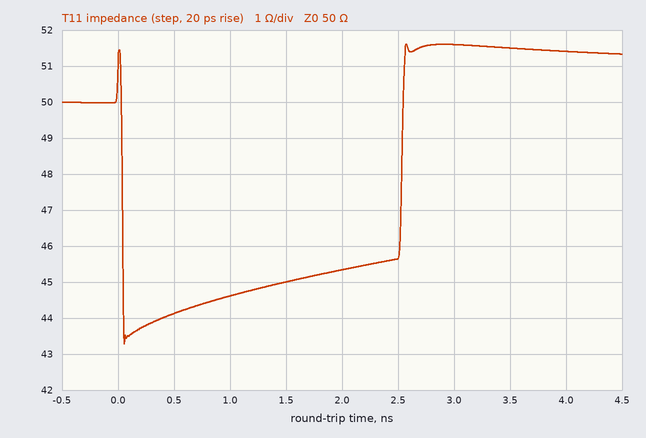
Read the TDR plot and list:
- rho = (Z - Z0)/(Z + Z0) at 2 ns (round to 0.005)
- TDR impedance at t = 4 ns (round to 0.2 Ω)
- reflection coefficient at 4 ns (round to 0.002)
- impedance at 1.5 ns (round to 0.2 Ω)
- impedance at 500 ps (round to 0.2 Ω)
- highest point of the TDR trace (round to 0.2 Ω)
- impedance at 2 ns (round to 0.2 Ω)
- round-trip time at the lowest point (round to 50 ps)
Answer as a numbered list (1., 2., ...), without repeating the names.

1. -0.050
2. 51.4 Ω
3. +0.014
4. 45.0 Ω
5. 44.2 Ω
6. 51.6 Ω
7. 45.4 Ω
8. 50 ps
